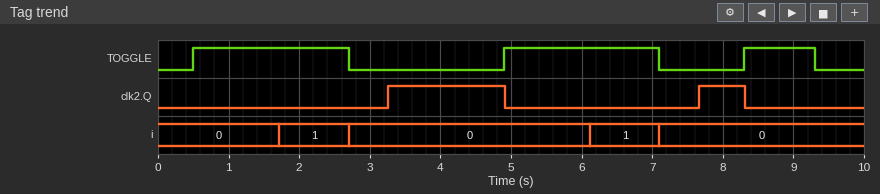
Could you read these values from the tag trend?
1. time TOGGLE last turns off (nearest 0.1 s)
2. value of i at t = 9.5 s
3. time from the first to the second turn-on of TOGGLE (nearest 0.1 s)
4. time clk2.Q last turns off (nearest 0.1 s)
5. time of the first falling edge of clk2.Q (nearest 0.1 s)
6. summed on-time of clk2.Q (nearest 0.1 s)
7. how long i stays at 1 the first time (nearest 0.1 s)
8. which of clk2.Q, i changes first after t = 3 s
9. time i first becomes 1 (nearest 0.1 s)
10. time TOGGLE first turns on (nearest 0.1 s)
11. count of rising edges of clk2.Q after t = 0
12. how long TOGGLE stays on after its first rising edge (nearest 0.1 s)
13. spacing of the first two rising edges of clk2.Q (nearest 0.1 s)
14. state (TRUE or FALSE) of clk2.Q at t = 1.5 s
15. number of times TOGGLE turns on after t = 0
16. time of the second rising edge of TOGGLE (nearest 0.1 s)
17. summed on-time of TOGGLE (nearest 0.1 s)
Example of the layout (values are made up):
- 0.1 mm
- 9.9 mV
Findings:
- 9.3 s
- 0
- 4.4 s
- 8.3 s
- 4.9 s
- 2.3 s
- 1.0 s
- clk2.Q
- 1.7 s
- 0.5 s
- 2
- 2.2 s
- 4.4 s
- FALSE
- 3
- 4.9 s
- 5.4 s
